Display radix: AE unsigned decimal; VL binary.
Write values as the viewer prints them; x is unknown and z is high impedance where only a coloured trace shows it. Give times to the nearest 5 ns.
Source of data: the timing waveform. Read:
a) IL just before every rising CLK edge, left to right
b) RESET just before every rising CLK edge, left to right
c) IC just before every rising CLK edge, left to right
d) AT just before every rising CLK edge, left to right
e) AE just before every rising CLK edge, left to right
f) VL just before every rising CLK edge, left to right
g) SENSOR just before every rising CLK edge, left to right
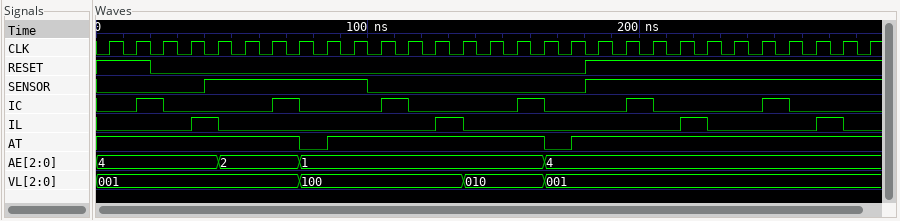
0 0 0 0 1 0 0 0 0 0 0 0 0 1 0 0 0 0 0 0 0 0 1 0 0 0 0 1 0
1 1 0 0 0 0 0 0 0 0 0 0 0 0 0 0 0 0 1 1 1 1 1 1 1 1 1 1 1
0 0 1 0 0 0 0 1 0 0 0 1 0 0 0 0 1 0 0 0 1 0 0 0 0 1 0 0 0
1 1 1 1 1 1 1 1 0 1 1 1 1 1 1 1 1 0 1 1 1 1 1 1 1 1 1 1 1
4, 4, 4, 4, 4, 2, 2, 2, 1, 1, 1, 1, 1, 1, 1, 1, 1, 4, 4, 4, 4, 4, 4, 4, 4, 4, 4, 4, 4
001, 001, 001, 001, 001, 001, 001, 001, 100, 100, 100, 100, 100, 100, 010, 010, 010, 001, 001, 001, 001, 001, 001, 001, 001, 001, 001, 001, 001
0 0 0 0 1 1 1 1 1 1 0 0 0 0 0 0 0 0 1 1 1 1 1 1 1 1 1 1 1
